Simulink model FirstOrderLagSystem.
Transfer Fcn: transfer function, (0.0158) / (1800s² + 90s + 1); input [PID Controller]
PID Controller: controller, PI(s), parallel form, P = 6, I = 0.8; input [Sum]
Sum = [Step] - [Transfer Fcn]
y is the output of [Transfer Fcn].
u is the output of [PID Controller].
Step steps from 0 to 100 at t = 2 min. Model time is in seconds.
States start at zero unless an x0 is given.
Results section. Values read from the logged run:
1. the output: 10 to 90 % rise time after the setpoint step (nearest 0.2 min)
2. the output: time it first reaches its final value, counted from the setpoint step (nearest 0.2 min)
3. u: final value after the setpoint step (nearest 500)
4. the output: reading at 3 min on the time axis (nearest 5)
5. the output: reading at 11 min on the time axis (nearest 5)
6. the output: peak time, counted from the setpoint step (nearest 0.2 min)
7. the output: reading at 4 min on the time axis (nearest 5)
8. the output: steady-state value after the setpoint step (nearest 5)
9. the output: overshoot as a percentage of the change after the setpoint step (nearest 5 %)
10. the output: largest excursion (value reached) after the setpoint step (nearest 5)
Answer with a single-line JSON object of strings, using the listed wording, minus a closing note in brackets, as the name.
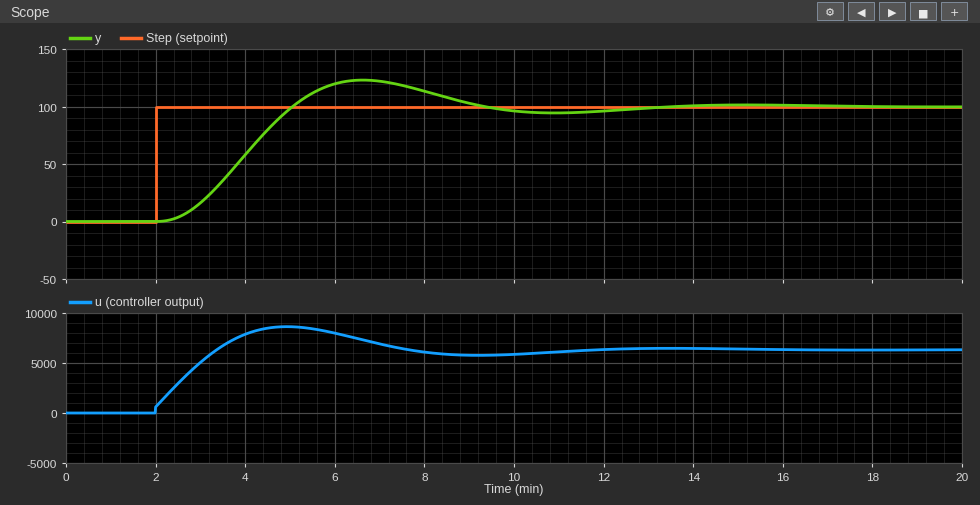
{"the output: 10 to 90 % rise time after the setpoint step": "2.0 min", "the output: time it first reaches its final value, counted from the setpoint step": "3.0 min", "u: final value after the setpoint step": "6500", "the output: reading at 3 min on the time axis": "15", "the output: reading at 11 min on the time axis": "95", "the output: peak time, counted from the setpoint step": "4.6 min", "the output: reading at 4 min on the time axis": "60", "the output: steady-state value after the setpoint step": "100", "the output: overshoot as a percentage of the change after the setpoint step": "25 %", "the output: largest excursion (value reached) after the setpoint step": "125"}
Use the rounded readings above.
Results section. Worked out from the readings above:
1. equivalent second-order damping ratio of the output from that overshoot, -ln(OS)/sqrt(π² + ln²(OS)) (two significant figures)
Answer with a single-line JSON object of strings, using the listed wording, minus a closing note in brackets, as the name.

{"equivalent second-order damping ratio of the output from that overshoot, -ln(OS)/sqrt(π² + ln²(OS))": "0.40"}
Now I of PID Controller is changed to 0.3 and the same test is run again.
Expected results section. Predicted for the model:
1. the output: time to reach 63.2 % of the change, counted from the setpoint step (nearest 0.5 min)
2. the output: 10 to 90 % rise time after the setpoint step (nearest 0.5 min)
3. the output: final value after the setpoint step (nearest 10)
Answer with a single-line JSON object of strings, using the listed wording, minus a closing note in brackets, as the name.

{"the output: time to reach 63.2 % of the change, counted from the setpoint step": "4.0 min", "the output: 10 to 90 % rise time after the setpoint step": "5.5 min", "the output: final value after the setpoint step": "100"}
